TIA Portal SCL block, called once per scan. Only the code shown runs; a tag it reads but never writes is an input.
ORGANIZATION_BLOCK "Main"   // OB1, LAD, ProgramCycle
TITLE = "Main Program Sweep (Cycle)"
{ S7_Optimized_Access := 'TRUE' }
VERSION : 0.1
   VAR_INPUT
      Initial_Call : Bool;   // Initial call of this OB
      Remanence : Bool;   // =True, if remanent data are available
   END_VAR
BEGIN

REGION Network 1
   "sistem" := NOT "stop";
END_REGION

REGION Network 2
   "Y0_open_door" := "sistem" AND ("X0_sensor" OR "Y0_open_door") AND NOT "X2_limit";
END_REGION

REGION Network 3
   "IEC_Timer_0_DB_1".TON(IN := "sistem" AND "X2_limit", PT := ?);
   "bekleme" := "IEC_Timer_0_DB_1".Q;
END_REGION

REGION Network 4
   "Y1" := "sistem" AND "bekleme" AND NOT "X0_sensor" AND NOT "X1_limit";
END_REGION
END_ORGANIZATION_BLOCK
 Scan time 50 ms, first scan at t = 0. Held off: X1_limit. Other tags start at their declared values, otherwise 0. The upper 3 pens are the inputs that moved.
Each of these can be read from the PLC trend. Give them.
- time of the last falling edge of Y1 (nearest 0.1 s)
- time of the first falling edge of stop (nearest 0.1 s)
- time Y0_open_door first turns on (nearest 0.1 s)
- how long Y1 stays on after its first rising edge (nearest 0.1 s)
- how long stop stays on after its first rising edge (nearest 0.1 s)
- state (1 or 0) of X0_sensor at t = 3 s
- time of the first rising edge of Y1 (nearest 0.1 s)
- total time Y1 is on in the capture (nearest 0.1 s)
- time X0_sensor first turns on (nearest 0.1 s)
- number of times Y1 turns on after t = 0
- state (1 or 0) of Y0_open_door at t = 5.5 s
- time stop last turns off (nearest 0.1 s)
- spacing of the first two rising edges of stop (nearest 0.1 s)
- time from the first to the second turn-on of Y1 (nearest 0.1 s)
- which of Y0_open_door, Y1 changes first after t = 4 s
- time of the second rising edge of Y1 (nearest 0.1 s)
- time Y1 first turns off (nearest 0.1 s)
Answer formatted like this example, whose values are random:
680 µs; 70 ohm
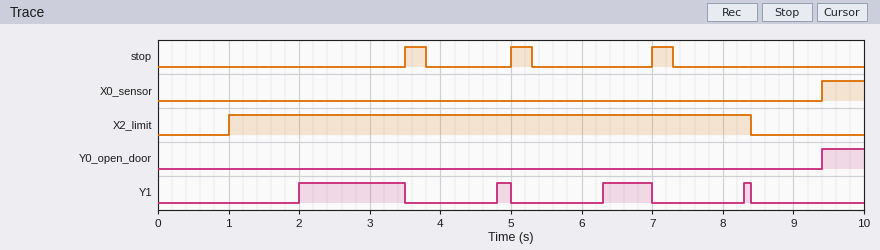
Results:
8.4 s; 3.8 s; 9.4 s; 1.5 s; 0.3 s; 0; 2.0 s; 2.5 s; 9.4 s; 4; 0; 7.3 s; 1.5 s; 2.8 s; Y1; 4.8 s; 3.5 s
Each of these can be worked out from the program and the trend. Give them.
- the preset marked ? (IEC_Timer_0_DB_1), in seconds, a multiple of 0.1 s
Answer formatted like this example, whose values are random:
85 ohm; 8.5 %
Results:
1.0 s
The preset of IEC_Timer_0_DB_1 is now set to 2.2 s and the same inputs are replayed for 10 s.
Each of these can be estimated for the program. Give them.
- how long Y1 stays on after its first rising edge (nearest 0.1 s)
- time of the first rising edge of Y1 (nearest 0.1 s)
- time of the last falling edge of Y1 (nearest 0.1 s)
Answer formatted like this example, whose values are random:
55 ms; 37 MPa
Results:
0.3 s; 3.2 s; 3.5 s
